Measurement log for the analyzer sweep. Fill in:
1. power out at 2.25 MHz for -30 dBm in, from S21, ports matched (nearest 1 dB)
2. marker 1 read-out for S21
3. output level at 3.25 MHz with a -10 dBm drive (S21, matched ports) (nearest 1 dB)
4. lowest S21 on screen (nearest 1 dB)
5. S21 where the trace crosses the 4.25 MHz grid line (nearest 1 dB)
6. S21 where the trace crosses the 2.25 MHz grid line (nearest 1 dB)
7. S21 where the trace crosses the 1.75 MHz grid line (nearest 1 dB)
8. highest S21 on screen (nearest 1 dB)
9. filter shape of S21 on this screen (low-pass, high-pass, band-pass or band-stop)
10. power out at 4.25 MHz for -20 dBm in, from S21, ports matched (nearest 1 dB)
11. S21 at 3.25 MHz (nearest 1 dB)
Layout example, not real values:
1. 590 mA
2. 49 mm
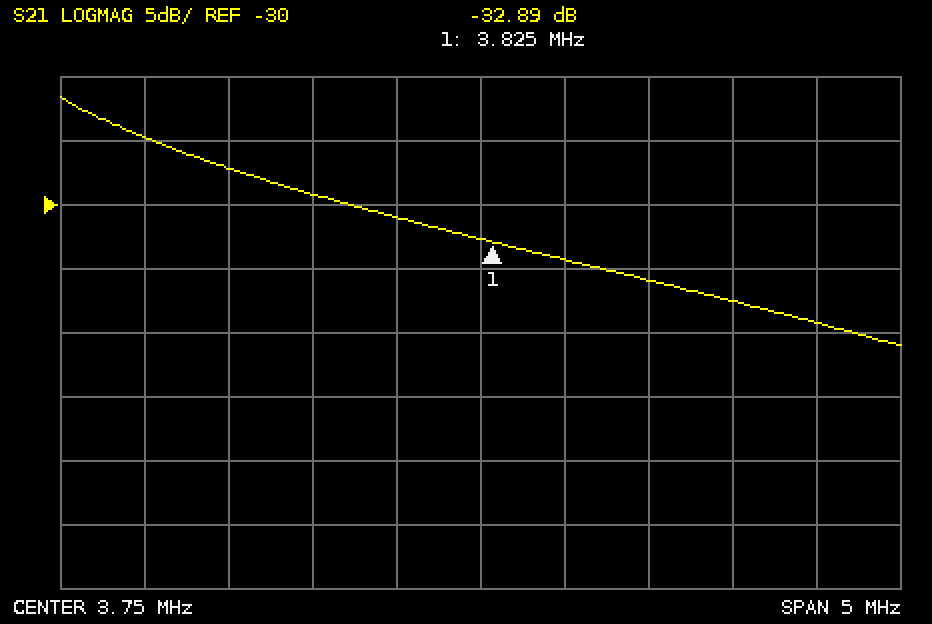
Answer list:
1. -57 dBm
2. -32.89 dB
3. -41 dBm
4. -41 dB
5. -34 dB
6. -27 dB
7. -25 dB
8. -22 dB
9. low-pass
10. -54 dBm
11. -31 dB
